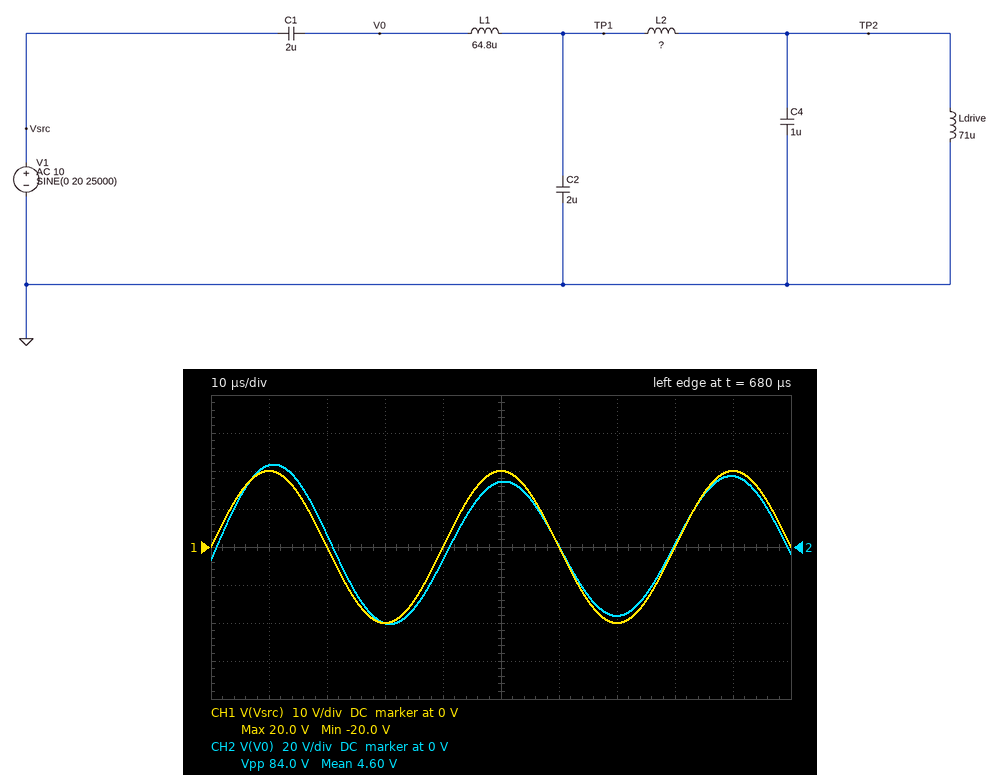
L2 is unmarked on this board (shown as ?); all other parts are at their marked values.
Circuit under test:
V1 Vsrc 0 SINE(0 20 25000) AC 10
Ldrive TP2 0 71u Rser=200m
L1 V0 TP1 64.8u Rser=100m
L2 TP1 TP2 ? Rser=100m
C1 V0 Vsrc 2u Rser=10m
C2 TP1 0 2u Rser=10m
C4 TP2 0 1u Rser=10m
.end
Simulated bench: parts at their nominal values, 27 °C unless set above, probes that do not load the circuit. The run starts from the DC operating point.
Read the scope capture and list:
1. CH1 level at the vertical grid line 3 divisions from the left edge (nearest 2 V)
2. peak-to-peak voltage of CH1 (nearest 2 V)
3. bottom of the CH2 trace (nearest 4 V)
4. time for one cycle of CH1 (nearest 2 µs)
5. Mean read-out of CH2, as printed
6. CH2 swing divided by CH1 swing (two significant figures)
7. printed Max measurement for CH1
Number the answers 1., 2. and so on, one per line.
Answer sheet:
1. -20 V
2. 40 V
3. -40 V
4. 40 µs
5. 4.60 V
6. 2.1
7. 20.0 V
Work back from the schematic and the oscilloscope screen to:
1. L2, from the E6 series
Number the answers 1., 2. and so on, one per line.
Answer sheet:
1. 220 µH
